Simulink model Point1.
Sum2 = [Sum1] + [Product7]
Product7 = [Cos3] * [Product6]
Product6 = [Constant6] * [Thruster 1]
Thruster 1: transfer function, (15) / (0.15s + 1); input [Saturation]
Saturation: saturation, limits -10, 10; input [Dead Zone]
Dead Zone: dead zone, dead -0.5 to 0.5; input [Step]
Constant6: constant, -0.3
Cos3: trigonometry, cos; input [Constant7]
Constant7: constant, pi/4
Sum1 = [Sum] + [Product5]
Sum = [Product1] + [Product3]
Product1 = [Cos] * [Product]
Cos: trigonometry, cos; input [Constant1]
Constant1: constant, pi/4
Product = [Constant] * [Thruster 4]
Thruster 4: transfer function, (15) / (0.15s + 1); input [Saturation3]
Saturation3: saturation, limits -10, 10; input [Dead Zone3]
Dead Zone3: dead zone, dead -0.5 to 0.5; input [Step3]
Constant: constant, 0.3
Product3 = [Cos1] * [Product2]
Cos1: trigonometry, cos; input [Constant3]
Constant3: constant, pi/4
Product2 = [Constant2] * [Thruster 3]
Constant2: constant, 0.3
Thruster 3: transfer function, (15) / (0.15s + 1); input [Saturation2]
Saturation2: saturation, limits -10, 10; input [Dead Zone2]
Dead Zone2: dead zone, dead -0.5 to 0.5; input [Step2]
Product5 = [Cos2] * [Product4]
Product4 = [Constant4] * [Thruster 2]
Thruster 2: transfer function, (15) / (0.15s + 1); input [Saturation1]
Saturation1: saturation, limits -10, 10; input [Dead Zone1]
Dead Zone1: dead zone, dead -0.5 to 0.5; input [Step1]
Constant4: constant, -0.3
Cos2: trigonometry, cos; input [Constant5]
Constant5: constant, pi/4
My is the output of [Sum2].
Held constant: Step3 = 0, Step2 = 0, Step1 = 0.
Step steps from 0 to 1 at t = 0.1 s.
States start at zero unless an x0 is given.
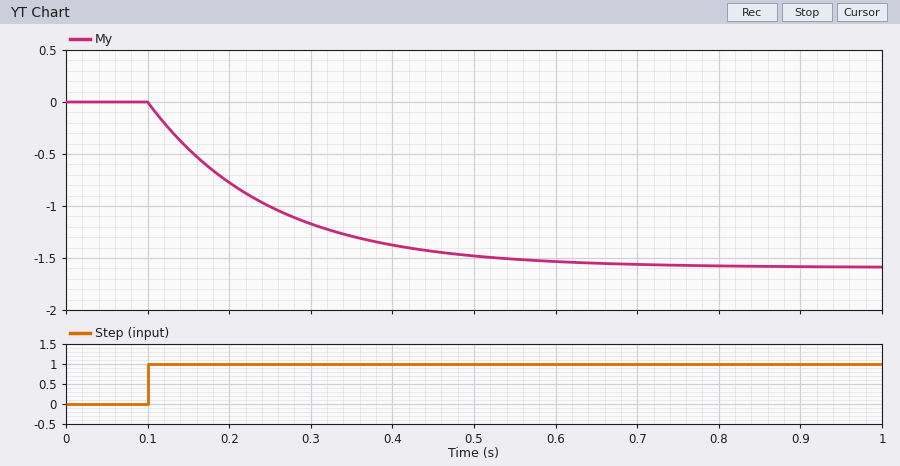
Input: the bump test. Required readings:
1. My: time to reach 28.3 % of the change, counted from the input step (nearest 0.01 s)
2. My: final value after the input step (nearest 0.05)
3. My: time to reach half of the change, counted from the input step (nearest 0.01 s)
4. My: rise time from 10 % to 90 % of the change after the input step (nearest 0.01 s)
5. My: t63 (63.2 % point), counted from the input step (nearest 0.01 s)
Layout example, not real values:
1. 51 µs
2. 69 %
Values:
1. 0.05 s
2. -1.60
3. 0.10 s
4. 0.33 s
5. 0.15 s
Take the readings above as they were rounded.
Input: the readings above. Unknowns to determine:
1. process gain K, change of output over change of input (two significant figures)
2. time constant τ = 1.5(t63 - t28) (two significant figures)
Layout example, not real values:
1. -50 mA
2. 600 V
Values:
1. -1.6
2. 0.15 s
